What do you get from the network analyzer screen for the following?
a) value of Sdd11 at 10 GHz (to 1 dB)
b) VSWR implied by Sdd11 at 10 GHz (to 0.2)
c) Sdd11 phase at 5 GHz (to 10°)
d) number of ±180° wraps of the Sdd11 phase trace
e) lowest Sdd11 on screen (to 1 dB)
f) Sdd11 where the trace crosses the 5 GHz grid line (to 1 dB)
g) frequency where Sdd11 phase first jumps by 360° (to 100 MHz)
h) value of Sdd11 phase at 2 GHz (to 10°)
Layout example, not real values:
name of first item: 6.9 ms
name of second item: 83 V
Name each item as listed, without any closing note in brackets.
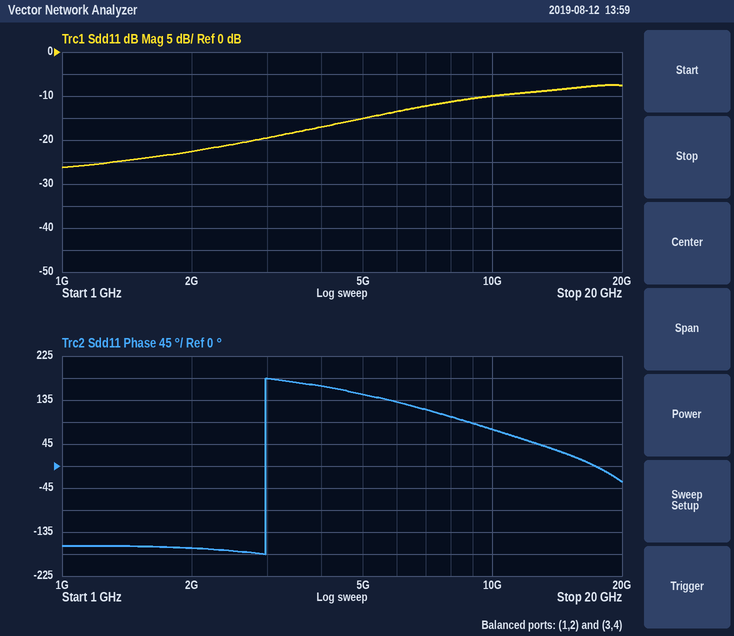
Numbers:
value of Sdd11 at 10 GHz: -10 dB
VSWR implied by Sdd11 at 10 GHz: 2.0
Sdd11 phase at 5 GHz: 150°
number of ±180° wraps of the Sdd11 phase trace: 1
lowest Sdd11 on screen: -26 dB
Sdd11 where the trace crosses the 5 GHz grid line: -15 dB
frequency where Sdd11 phase first jumps by 360°: 3.0 GHz
value of Sdd11 phase at 2 GHz: -170°
